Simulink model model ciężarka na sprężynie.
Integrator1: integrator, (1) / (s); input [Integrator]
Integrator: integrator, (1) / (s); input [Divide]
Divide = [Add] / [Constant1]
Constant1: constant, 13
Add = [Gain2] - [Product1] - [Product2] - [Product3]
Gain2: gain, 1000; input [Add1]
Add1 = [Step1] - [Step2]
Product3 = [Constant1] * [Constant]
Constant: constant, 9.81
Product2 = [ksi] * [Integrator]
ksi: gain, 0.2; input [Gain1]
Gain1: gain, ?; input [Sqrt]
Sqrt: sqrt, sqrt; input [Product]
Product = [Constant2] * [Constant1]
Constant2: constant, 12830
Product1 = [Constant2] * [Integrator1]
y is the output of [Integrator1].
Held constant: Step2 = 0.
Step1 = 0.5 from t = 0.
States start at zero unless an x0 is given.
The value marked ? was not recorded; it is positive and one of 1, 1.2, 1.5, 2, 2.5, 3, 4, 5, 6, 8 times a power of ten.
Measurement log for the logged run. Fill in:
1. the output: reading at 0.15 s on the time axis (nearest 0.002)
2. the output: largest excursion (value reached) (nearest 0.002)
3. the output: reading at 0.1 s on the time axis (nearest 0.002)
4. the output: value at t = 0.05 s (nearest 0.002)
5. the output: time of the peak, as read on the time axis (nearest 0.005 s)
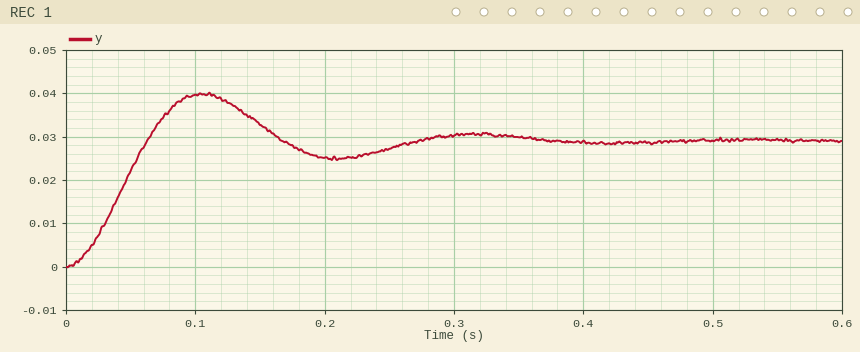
0.032
0.040
0.040
0.022
0.105 s
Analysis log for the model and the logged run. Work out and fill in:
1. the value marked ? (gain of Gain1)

3
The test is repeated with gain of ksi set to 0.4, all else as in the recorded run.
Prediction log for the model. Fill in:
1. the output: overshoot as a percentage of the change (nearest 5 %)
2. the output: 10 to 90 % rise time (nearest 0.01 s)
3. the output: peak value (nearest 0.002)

10 %
0.06 s
0.032
